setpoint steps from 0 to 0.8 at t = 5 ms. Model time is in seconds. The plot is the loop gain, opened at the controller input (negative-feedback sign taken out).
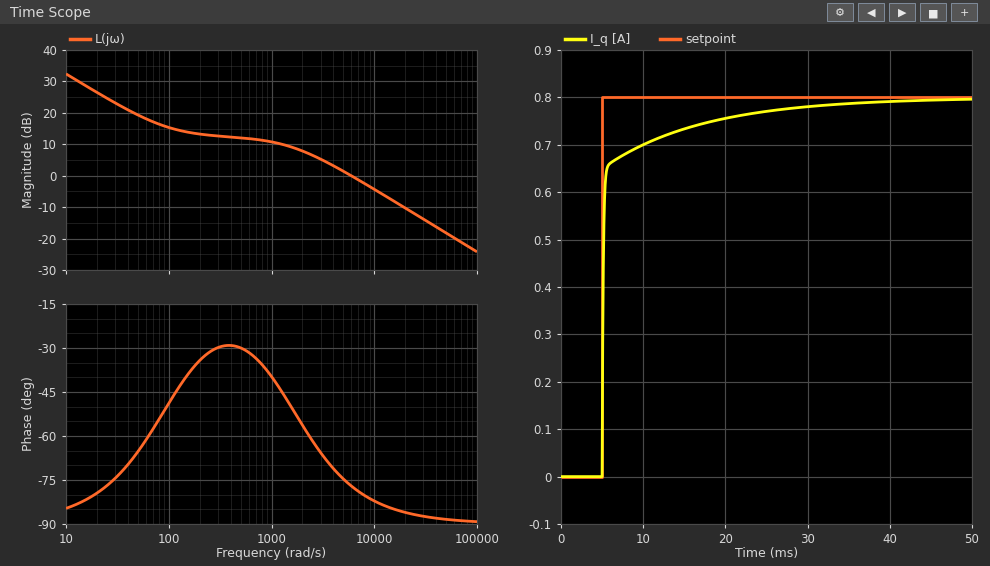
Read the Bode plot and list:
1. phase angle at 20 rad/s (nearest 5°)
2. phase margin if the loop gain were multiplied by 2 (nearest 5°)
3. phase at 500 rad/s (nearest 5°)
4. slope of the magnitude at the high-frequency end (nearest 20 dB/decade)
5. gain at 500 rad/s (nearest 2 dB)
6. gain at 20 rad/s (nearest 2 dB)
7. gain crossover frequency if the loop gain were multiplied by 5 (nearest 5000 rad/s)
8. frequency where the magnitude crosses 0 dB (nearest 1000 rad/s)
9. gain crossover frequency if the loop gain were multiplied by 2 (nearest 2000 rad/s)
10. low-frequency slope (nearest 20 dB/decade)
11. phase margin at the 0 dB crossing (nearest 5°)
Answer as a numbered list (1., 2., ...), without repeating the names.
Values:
1. -80°
2. 95°
3. -30°
4. -20 dB/decade
5. 12 dB
6. 26 dB
7. 30000 rad/s
8. 6000 rad/s
9. 12000 rad/s
10. -20 dB/decade
11. 105°
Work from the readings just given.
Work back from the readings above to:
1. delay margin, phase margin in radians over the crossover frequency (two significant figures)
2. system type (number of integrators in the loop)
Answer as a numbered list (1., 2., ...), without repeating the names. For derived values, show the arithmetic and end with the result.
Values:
1. 105 × π / 180 / 6000 = 0.00031 s
2. 1
